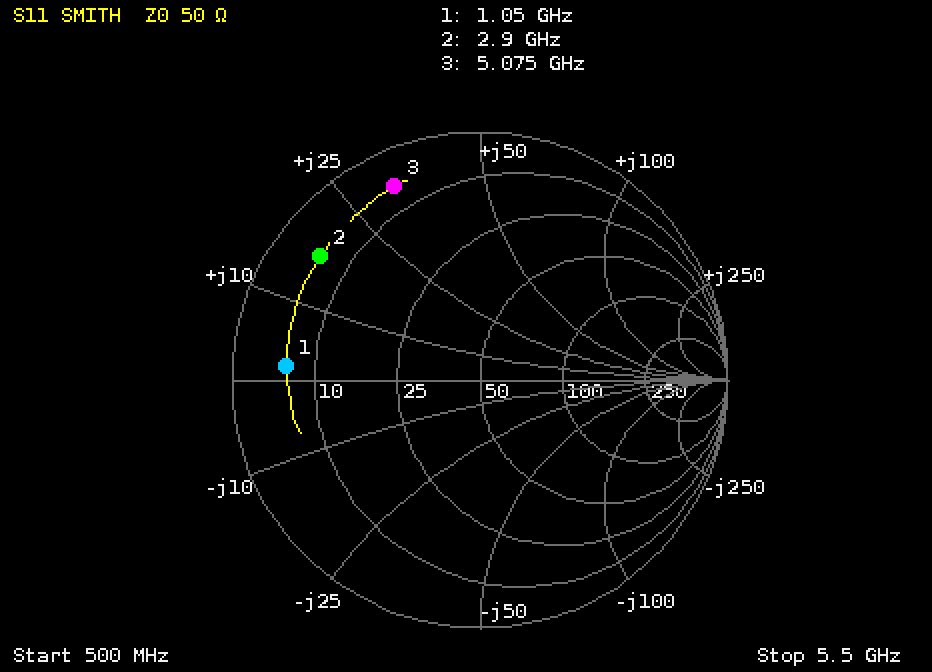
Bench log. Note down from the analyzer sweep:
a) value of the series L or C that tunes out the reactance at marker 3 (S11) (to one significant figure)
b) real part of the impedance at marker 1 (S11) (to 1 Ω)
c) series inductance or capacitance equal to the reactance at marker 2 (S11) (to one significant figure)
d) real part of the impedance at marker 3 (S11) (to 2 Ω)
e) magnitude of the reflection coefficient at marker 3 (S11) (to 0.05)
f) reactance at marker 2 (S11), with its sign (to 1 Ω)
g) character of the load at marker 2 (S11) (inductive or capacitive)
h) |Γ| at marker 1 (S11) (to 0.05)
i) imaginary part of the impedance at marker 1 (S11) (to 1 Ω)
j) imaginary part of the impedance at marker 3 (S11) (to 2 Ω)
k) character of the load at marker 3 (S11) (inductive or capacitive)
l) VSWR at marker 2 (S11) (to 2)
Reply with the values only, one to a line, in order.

1.0 pF
6 Ω
900 pH
6 Ω
0.85
+17 Ω
inductive
0.80
+2 Ω
+32 Ω
inductive
10
